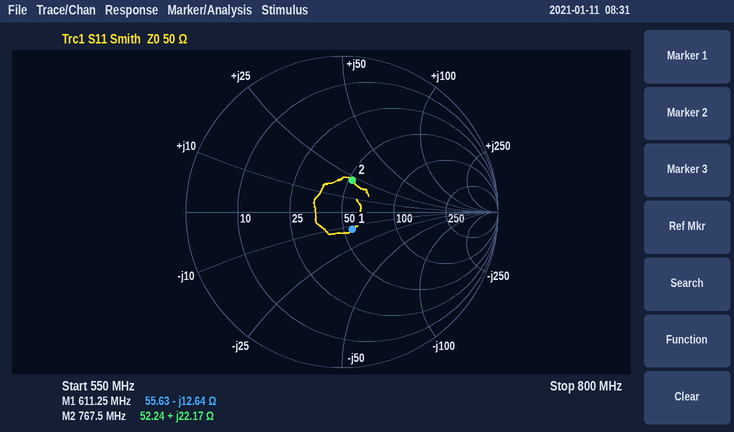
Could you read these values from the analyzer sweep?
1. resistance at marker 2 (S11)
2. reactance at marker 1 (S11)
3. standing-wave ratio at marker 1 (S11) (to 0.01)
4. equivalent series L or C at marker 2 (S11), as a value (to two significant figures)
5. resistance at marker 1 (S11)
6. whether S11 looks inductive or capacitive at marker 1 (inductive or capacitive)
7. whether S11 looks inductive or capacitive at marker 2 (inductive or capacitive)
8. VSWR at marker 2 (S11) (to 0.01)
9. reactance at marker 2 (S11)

52.24 Ω
-12.64 Ω
1.30
4.6 nH
55.63 Ω
capacitive
inductive
1.54
+22.17 Ω
